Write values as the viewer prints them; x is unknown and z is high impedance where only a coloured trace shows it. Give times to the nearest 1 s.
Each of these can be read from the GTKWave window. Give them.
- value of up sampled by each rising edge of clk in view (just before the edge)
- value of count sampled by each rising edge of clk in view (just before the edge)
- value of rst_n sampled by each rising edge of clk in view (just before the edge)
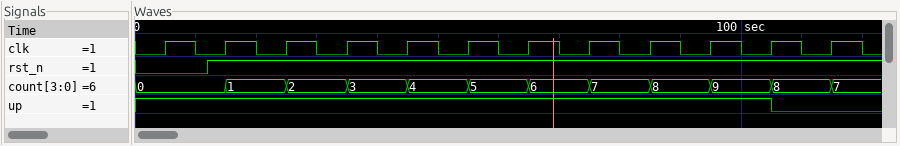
1 1 1 1 1 1 1 1 1 1 1 0
0, 0, 1, 2, 3, 4, 5, 6, 7, 8, 9, 8
0 1 1 1 1 1 1 1 1 1 1 1
